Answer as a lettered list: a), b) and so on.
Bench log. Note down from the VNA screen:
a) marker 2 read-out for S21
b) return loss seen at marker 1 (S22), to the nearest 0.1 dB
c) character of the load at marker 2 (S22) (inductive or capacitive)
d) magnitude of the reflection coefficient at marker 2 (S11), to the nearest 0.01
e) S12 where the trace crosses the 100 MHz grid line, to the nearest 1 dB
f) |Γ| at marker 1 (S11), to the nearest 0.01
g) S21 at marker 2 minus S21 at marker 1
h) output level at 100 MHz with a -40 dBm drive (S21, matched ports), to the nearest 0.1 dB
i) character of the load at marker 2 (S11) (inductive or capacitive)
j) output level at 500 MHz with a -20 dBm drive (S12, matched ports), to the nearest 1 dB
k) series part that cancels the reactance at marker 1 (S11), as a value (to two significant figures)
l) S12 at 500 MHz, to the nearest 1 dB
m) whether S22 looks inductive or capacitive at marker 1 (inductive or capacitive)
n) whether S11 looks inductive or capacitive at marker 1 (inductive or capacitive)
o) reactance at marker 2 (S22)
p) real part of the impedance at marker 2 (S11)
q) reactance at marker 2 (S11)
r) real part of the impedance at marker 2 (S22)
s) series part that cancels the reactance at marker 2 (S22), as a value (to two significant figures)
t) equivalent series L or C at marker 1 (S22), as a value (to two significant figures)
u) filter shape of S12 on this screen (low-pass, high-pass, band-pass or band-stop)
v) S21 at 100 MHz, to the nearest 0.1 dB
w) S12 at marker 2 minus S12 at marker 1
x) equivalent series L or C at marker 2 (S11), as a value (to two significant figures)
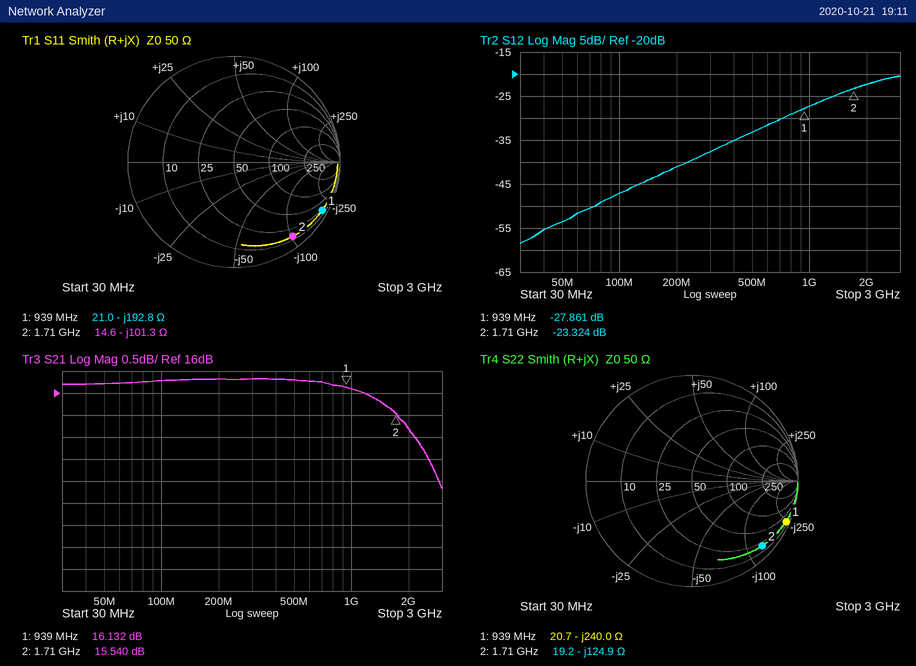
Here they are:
a) 15.540 dB
b) 0.3 dB
c) capacitive
d) 0.89
e) -47 dB
f) 0.95
g) -0.592 dB
h) -23.7 dBm
i) capacitive
j) -53 dBm
k) 33 nH
l) -33 dB
m) capacitive
n) capacitive
o) -124.9 Ω
p) 14.6 Ω
q) -101.3 Ω
r) 19.2 Ω
s) 12 nH
t) 710 fF
u) high-pass
v) 16.3 dB
w) 4.537 dB
x) 920 fF
